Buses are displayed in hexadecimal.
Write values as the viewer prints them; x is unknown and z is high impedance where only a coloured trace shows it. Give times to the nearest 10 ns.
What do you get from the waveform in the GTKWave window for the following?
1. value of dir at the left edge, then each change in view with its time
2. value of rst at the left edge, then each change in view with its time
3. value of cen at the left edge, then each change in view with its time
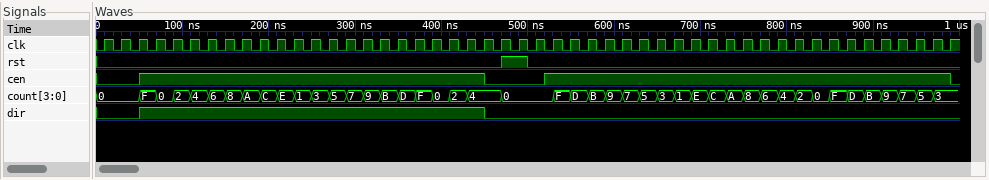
0, 1 at 50 ns, 0 at 450 ns
0, 1 at 470 ns, 0 at 500 ns
0, 1 at 50 ns, 0 at 450 ns, 1 at 520 ns, 0 at 990 ns
